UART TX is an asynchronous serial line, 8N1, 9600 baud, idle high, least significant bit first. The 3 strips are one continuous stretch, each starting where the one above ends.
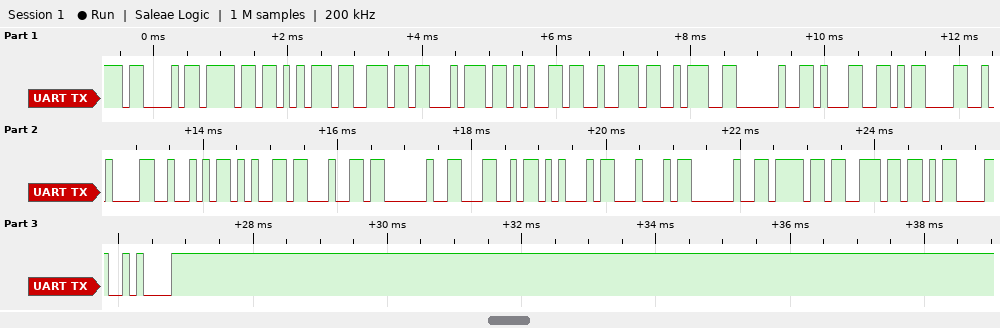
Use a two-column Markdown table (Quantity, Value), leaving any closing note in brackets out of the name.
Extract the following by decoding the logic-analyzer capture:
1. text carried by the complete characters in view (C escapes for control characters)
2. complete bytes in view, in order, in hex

| Quantity | Value |
|---|---|
| text carried by the complete characters in view | "Counter: 1\r\nRed LED on\r\n" |
| complete bytes in view, in order, in hex | 43 6F 75 6E 74 65 72 3A 20 31 0D 0A 52 65 64 20 4C 45 44 20 6F 6E 0D 0A |
